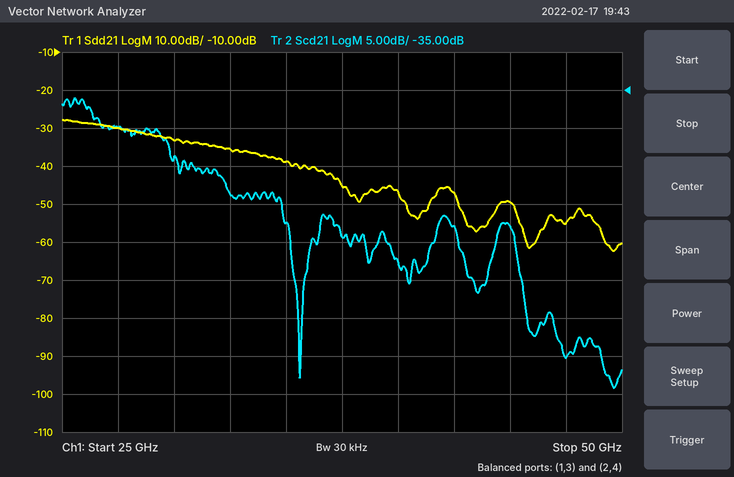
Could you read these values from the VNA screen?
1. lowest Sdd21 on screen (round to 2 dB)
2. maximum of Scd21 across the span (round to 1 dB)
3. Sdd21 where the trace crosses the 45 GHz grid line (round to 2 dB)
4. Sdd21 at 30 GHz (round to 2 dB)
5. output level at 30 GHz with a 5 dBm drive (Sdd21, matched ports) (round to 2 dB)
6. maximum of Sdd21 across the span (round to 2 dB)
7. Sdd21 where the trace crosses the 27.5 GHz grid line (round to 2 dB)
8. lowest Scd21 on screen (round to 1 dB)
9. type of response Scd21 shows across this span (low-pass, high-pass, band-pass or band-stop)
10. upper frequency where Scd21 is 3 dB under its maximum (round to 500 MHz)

-62 dB
-36 dB
-50 dB
-34 dB
-28 dBm
-28 dB
-30 dB
-74 dB
low-pass
26.5 GHz
